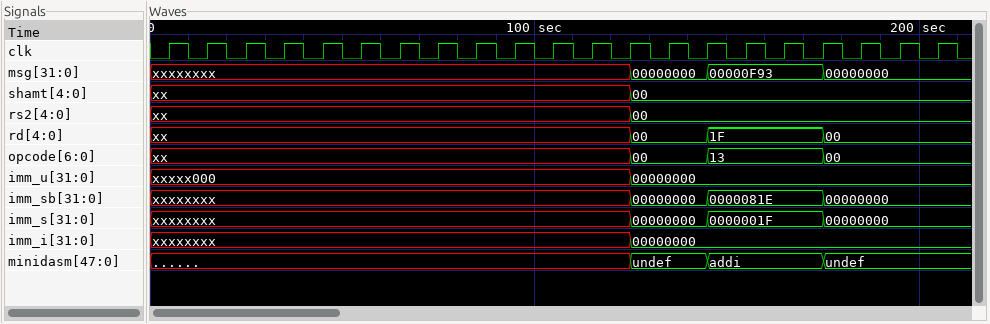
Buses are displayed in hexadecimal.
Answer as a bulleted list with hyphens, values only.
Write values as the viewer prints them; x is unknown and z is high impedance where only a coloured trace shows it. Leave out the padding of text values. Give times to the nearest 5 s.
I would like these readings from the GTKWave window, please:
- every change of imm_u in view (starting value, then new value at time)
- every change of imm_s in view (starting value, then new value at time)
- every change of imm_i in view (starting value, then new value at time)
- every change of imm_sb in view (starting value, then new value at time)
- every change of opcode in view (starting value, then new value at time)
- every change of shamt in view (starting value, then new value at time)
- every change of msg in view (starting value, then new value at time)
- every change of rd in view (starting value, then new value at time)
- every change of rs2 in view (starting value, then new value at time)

- xxxxx000, 00000000 at 125 s
- xxxxxxxx, 00000000 at 125 s, 0000001F at 145 s, 00000000 at 175 s
- xxxxxxxx, 00000000 at 125 s
- xxxxxxxx, 00000000 at 125 s, 0000081E at 145 s, 00000000 at 175 s
- xx, 00 at 125 s, 13 at 145 s, 00 at 175 s
- xx, 00 at 125 s
- xxxxxxxx, 00000000 at 125 s, 00000F93 at 145 s, 00000000 at 175 s
- xx, 00 at 125 s, 1F at 145 s, 00 at 175 s
- xx, 00 at 125 s
